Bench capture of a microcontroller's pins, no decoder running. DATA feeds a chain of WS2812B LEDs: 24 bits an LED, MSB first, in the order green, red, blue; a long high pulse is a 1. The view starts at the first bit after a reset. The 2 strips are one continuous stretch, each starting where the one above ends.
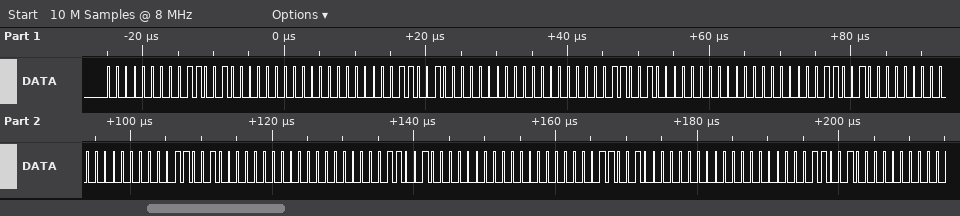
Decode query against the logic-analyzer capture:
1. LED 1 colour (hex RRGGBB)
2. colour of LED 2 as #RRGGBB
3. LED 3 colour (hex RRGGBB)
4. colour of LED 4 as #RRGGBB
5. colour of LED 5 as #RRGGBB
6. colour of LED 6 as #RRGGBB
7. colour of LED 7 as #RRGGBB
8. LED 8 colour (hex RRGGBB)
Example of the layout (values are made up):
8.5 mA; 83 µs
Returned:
#640000; #640000; #640000; #640000; #640000; #640000; #640000; #640000
